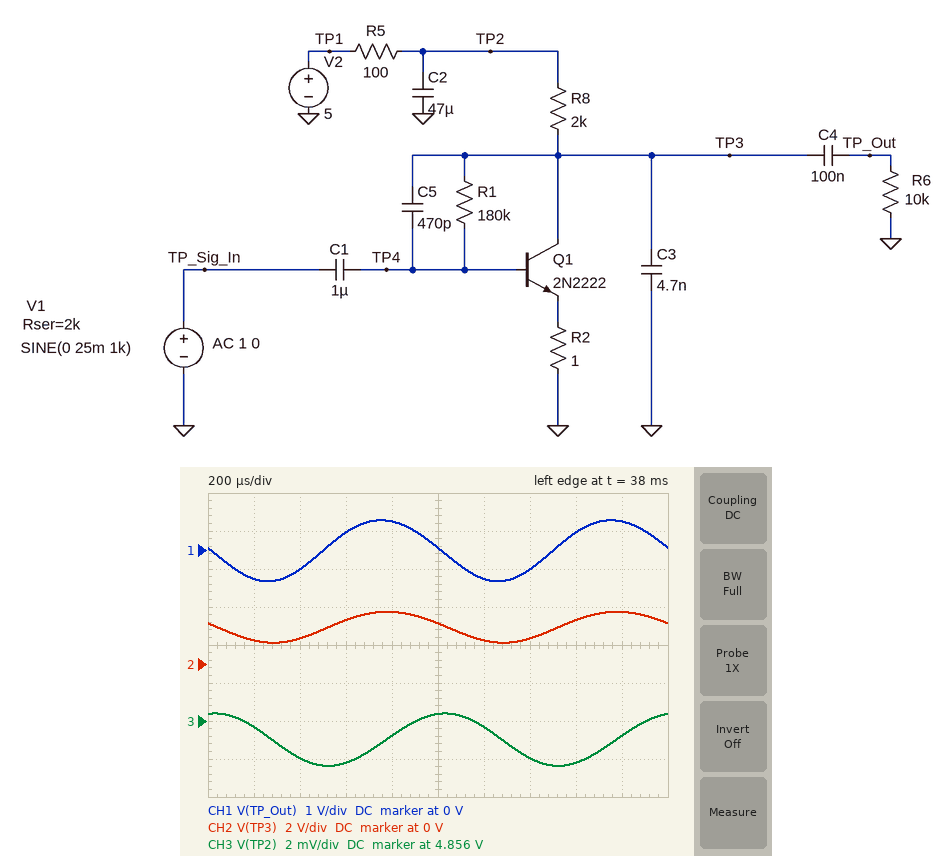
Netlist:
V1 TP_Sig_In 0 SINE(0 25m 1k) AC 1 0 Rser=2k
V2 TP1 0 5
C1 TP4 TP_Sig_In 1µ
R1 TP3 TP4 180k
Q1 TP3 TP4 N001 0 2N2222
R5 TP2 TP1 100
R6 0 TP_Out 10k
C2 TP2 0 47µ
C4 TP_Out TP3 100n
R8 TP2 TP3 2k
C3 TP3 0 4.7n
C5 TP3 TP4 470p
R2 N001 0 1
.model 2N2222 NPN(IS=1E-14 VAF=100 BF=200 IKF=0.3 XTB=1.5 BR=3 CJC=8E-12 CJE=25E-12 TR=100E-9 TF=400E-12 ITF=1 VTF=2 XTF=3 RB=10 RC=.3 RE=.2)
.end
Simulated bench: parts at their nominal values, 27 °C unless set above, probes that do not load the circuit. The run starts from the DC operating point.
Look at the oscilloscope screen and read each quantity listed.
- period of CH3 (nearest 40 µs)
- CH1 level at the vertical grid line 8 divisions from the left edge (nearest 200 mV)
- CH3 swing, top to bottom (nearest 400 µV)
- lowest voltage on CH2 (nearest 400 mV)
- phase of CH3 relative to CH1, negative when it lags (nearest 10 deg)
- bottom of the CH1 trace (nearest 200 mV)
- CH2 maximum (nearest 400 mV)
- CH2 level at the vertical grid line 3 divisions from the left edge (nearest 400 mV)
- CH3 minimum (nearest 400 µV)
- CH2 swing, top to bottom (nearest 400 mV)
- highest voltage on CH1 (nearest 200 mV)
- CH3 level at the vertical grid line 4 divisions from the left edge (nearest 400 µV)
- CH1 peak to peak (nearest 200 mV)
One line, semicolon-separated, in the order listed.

1.00 ms; 400 mV; 2.8 mV; 1.2 V; -100 deg; -800 mV; 2.8 V; 2.4 V; 4.8536 V; 1.6 V; 800 mV; 4.8552 V; 1.6 V
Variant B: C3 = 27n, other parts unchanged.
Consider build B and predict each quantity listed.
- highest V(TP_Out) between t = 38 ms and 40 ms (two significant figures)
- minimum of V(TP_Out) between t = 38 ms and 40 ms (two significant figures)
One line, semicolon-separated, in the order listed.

750 mV; -790 mV
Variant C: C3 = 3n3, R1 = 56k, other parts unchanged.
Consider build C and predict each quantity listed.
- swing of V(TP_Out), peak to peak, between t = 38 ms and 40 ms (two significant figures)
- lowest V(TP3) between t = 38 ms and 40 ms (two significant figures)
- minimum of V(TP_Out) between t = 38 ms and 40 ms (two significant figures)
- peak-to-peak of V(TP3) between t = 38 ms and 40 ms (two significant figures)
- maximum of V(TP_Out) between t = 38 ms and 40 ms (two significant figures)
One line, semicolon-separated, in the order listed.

930 mV; 710 mV; -470 mV; 940 mV; 460 mV
